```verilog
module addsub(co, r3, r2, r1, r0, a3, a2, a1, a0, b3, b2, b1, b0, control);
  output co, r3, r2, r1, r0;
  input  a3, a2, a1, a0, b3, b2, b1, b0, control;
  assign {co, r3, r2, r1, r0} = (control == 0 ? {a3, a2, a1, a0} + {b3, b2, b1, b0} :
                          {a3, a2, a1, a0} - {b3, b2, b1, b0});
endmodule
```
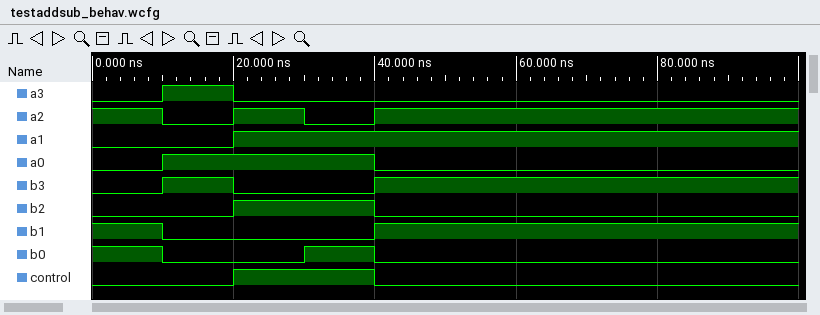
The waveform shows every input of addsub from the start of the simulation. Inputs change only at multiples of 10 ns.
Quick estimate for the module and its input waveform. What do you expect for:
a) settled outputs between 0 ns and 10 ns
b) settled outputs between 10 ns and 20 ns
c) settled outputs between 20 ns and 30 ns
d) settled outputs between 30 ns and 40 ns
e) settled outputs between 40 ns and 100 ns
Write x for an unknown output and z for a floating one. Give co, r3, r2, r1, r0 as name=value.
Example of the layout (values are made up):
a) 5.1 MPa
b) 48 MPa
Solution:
a) co=0, r3=0, r2=1, r1=1, r0=1
b) co=1, r3=0, r2=0, r1=0, r0=1
c) co=0, r3=0, r2=0, r1=1, r0=1
d) co=1, r3=1, r2=1, r1=1, r0=0
e) co=1, r3=0, r2=0, r1=0, r0=0
